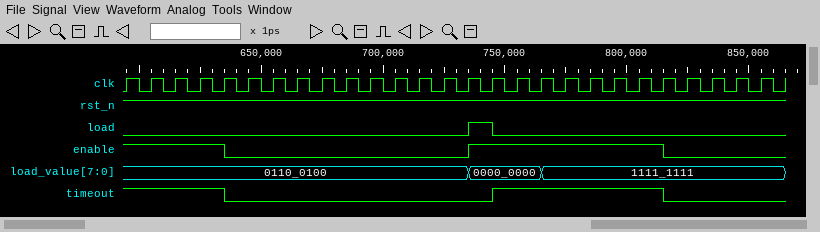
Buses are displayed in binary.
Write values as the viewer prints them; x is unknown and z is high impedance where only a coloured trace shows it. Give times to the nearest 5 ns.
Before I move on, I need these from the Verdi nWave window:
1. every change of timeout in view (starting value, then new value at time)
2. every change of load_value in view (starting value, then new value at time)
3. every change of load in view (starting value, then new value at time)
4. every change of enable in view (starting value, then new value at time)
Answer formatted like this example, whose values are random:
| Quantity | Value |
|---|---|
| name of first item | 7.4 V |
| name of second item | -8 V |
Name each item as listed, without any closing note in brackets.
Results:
| Quantity | Value |
|---|---|
| every change of timeout in view | 1, 0 at 635 ns, 1 at 745 ns, 0 at 815 ns |
| every change of load_value in view | 0110_0100, 0000_0000 at 735 ns, 1111_1111 at 765 ns |
| every change of load in view | 0, 1 at 735 ns, 0 at 745 ns |
| every change of enable in view | 1, 0 at 635 ns, 1 at 735 ns, 0 at 815 ns |
